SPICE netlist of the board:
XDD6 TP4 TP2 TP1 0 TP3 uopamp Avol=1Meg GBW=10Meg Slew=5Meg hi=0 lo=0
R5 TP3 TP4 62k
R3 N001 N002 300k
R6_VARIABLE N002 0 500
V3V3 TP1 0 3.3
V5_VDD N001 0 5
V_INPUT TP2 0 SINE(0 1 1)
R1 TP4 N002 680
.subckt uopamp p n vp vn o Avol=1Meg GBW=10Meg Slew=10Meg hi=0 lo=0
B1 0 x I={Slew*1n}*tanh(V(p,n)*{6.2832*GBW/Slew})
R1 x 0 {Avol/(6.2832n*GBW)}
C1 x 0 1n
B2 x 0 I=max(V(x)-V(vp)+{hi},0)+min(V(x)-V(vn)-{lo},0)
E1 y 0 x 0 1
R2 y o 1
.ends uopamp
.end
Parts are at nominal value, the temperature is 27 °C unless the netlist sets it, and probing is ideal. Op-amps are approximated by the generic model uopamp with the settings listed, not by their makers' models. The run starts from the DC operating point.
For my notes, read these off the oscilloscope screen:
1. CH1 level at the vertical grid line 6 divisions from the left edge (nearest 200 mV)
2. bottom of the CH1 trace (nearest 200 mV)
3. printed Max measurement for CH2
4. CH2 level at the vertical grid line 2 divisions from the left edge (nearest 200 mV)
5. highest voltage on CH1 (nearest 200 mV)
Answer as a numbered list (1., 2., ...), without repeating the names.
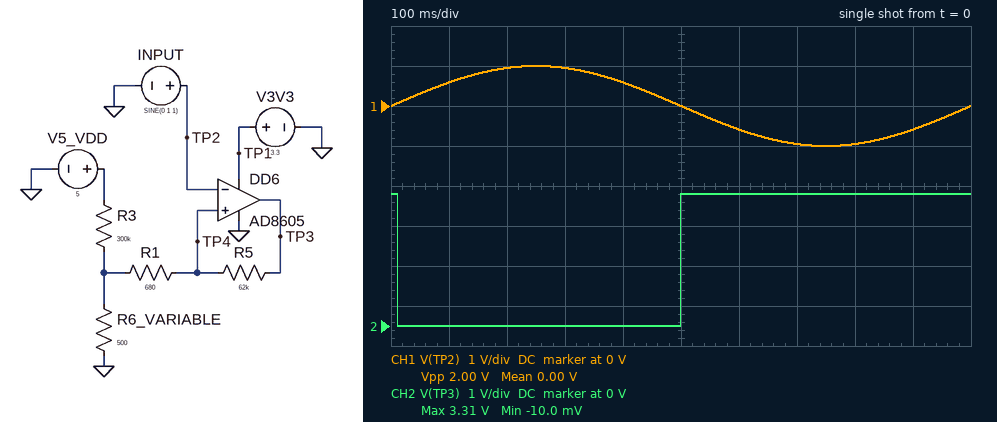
1. -600 mV
2. -1.0 V
3. 3.31 V
4. 0 V
5. 1.0 V
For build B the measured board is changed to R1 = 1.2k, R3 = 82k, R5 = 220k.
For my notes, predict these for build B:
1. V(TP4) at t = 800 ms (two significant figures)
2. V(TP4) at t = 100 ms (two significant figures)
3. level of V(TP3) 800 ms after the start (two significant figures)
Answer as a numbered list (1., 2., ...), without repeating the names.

1. 55 mV
2. 30 mV
3. 3.3 V
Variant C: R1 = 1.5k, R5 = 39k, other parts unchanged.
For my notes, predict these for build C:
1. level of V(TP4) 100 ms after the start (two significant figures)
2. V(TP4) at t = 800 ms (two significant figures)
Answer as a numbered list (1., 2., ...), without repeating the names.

1. 7.7 mV
2. 170 mV
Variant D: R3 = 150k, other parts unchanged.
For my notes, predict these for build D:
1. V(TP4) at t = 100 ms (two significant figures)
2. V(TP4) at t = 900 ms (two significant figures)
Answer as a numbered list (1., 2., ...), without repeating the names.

1. 16 mV
2. 78 mV
